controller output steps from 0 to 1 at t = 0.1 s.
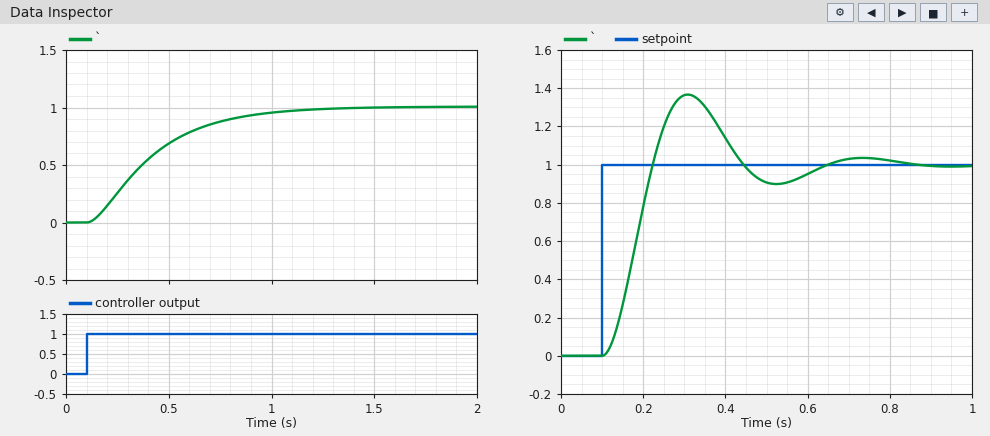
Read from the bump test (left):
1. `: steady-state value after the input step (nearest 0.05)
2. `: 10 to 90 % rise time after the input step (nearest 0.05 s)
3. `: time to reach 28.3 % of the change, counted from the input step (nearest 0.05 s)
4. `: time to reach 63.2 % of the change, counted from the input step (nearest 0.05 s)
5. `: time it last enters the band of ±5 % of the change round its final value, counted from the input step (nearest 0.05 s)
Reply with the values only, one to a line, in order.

1.00
0.65 s
0.15 s
0.35 s
0.90 s
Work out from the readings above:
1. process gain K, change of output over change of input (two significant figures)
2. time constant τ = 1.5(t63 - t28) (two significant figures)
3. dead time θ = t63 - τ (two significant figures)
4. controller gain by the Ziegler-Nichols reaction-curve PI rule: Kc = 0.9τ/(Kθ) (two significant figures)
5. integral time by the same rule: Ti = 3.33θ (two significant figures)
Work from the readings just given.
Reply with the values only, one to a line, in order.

1.0
0.30 s
0.050 s
5.4
0.17 s
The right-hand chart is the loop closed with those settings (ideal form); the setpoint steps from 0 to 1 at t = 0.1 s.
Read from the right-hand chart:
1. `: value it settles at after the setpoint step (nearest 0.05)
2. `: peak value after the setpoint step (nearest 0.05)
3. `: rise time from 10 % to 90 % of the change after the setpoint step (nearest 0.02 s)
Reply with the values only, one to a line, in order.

1.00
1.35
0.08 s
